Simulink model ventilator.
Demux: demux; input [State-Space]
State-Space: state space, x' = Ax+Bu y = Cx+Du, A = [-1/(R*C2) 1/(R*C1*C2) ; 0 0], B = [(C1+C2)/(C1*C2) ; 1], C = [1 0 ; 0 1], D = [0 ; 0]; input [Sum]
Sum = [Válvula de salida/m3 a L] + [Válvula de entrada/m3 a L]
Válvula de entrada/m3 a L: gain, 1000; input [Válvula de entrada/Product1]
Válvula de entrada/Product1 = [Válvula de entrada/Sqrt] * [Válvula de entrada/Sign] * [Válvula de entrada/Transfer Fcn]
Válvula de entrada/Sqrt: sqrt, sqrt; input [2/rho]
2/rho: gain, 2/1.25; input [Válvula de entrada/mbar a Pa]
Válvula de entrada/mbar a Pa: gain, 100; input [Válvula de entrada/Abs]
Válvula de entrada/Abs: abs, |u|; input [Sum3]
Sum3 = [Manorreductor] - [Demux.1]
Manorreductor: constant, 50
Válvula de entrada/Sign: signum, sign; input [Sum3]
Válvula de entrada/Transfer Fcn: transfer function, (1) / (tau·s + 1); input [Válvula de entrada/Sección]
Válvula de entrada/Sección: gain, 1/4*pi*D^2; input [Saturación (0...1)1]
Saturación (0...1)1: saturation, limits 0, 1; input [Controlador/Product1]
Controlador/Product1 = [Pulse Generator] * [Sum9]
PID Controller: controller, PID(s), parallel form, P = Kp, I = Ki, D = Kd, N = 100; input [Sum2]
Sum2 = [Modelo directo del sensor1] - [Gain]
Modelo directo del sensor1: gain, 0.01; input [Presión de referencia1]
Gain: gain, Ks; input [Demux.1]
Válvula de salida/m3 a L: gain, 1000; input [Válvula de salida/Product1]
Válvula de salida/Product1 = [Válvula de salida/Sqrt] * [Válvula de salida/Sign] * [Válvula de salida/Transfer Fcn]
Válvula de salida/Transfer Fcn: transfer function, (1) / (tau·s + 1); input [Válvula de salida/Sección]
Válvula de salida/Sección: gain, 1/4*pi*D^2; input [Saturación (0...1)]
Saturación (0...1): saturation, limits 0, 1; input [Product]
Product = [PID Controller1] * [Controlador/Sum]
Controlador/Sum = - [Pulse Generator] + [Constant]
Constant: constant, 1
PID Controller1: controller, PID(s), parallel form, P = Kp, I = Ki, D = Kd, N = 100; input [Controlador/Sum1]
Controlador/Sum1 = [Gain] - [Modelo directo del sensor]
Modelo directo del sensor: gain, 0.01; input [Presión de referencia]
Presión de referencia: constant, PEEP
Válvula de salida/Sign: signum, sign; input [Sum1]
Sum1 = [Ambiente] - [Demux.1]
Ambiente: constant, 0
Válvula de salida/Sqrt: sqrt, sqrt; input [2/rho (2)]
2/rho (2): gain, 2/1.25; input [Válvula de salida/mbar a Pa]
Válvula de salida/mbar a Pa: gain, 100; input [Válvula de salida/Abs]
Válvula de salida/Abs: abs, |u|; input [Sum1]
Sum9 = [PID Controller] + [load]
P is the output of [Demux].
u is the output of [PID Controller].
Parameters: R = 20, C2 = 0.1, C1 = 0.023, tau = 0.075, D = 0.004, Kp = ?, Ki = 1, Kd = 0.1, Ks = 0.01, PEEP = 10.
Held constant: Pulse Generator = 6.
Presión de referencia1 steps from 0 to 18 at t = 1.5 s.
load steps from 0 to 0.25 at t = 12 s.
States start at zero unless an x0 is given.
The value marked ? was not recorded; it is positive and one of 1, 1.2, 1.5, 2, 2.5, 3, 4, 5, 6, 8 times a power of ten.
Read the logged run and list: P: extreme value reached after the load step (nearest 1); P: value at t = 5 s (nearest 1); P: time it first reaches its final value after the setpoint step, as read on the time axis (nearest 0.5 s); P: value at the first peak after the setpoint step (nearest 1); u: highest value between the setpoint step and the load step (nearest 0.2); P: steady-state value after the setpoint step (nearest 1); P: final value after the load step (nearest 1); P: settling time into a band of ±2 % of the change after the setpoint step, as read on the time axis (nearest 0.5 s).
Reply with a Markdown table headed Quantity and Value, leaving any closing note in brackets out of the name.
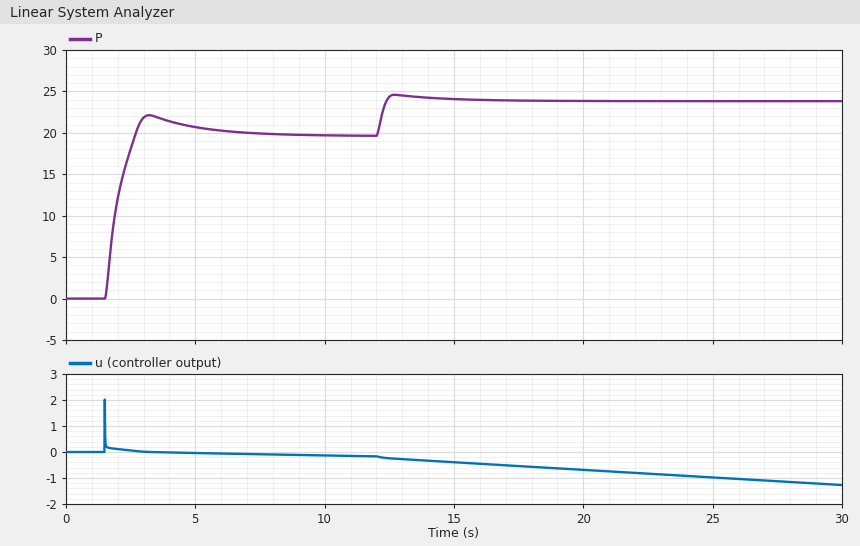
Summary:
| Quantity | Value |
|---|---|
| P: extreme value reached after the load step | 25 |
| P: value at t = 5 s | 21 |
| P: time it first reaches its final value after the setpoint step, as read on the time axis | 2.5 s |
| P: value at the first peak after the setpoint step | 22 |
| u: highest value between the setpoint step and the load step | 2.0 |
| P: steady-state value after the setpoint step | 20 |
| P: final value after the load step | 24 |
| P: settling time into a band of ±2 % of the change after the setpoint step, as read on the time axis | 7.0 s |
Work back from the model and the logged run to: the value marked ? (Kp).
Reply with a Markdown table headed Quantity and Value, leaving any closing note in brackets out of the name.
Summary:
| Quantity | Value |
|---|---|
| the value marked ? | 1.2 |
